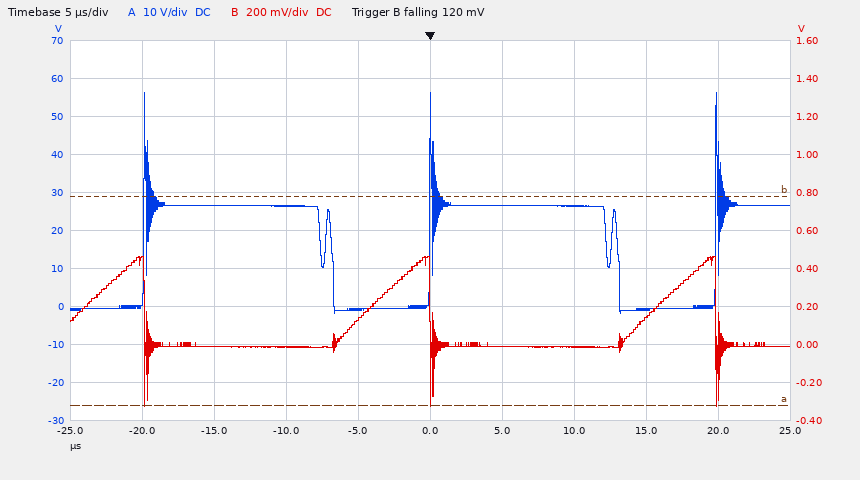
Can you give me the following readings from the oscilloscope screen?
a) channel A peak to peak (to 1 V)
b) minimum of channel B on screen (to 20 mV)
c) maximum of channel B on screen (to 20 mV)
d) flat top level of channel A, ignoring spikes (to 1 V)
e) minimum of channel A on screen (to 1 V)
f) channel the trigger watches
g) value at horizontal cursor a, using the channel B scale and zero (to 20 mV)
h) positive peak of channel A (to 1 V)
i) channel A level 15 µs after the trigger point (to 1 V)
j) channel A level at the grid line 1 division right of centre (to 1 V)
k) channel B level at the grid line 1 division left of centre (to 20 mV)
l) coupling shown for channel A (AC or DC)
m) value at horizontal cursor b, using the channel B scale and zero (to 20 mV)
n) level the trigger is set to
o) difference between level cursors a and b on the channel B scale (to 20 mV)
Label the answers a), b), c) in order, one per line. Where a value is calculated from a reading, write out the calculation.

a) 56 V − (-2 V) = 58 V
b) -320 mV
c) 460 mV
d) 27 V
e) -2 V
f) channel B
g) -320 mV
h) 56 V
i) -1 V
j) 27 V
k) 140 mV
l) DC
m) 780 mV
n) 120 mV
o) 1.10 V
